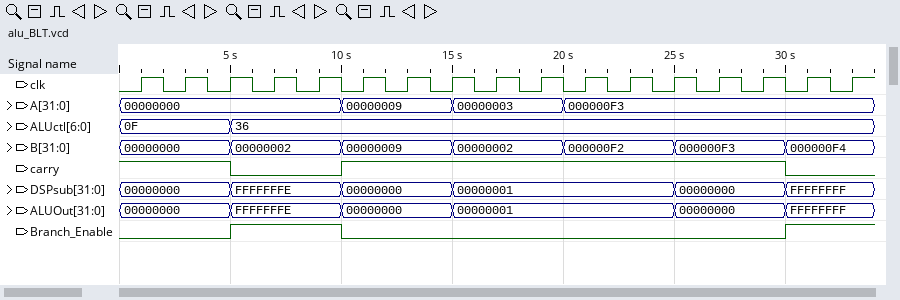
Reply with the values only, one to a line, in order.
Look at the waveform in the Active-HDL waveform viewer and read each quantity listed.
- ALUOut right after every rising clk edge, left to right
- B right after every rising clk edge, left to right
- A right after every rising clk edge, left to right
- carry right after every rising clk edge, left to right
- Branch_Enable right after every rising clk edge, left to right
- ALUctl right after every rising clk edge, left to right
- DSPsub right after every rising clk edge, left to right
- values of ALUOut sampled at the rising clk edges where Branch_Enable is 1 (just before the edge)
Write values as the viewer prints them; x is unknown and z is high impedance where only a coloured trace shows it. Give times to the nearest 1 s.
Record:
00000000, 00000000, FFFFFFFE, FFFFFFFE, FFFFFFFE, 00000000, 00000000, 00000001, 00000001, 00000001, 00000001, 00000001, 00000000, 00000000, 00000000, FFFFFFFF, FFFFFFFF
00000000, 00000000, 00000002, 00000002, 00000002, 00000009, 00000009, 00000002, 00000002, 00000002, 000000F2, 000000F2, 000000F3, 000000F3, 000000F3, 000000F4, 000000F4
00000000, 00000000, 00000000, 00000000, 00000000, 00000009, 00000009, 00000003, 00000003, 00000003, 000000F3, 000000F3, 000000F3, 000000F3, 000000F3, 000000F3, 000000F3
1 1 0 0 0 1 1 1 1 1 1 1 1 1 1 0 0
0 0 1 1 1 0 0 0 0 0 0 0 0 0 0 1 1
0F, 0F, 36, 36, 36, 36, 36, 36, 36, 36, 36, 36, 36, 36, 36, 36, 36
00000000, 00000000, FFFFFFFE, FFFFFFFE, FFFFFFFE, 00000000, 00000000, 00000001, 00000001, 00000001, 00000001, 00000001, 00000000, 00000000, 00000000, FFFFFFFF, FFFFFFFF
FFFFFFFE, FFFFFFFE, FFFFFFFF, FFFFFFFF
